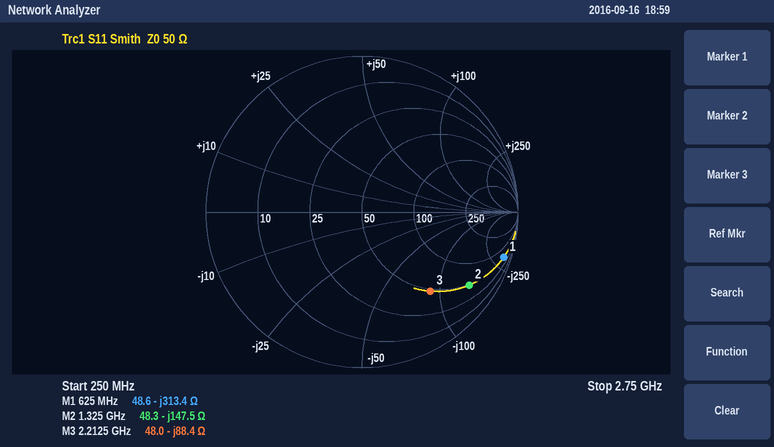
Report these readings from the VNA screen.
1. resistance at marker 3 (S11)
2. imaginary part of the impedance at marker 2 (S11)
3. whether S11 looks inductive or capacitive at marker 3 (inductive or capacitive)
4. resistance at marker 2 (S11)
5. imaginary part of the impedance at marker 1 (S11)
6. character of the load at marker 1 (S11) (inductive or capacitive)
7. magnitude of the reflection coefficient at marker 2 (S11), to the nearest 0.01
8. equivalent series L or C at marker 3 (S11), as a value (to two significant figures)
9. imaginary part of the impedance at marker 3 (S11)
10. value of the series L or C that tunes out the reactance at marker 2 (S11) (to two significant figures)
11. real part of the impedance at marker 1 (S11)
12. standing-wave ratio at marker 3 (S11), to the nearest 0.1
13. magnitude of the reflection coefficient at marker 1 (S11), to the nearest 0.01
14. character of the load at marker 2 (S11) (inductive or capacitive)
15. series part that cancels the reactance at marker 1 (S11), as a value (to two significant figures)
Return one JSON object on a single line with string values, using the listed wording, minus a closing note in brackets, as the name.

{"resistance at marker 3": "48.0 Ω", "imaginary part of the impedance at marker 2": "-147.5 Ω", "whether S11 looks inductive or capacitive at marker 3": "capacitive", "resistance at marker 2": "48.3 Ω", "imaginary part of the impedance at marker 1": "-313.4 Ω", "character of the load at marker 1 (S11)": "capacitive", "magnitude of the reflection coefficient at marker 2 (S11), to the nearest 0.01": "0.83", "equivalent series L or C at marker 3 (S11), as a value": "810 fF", "imaginary part of the impedance at marker 3": "-88.4 Ω", "value of the series L or C that tunes out the reactance at marker 2 (S11)": "18 nH", "real part of the impedance at marker 1": "48.6 Ω", "standing-wave ratio at marker 3 (S11), to the nearest 0.1": "5.1", "magnitude of the reflection coefficient at marker 1 (S11), to the nearest 0.01": "0.95", "character of the load at marker 2 (S11)": "capacitive", "series part that cancels the reactance at marker 1 (S11), as a value": "80 nH"}
